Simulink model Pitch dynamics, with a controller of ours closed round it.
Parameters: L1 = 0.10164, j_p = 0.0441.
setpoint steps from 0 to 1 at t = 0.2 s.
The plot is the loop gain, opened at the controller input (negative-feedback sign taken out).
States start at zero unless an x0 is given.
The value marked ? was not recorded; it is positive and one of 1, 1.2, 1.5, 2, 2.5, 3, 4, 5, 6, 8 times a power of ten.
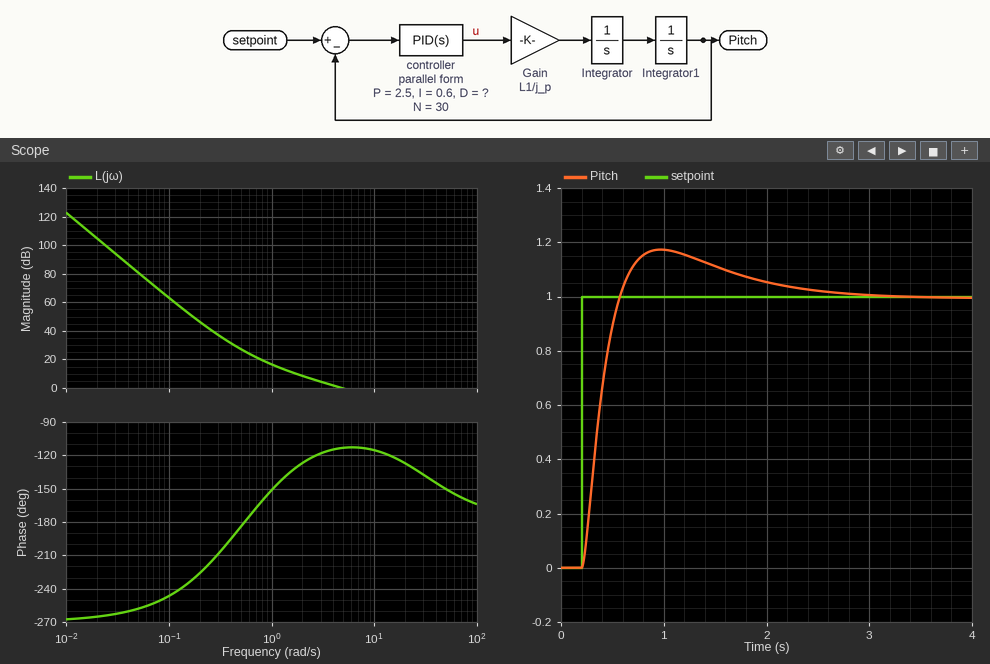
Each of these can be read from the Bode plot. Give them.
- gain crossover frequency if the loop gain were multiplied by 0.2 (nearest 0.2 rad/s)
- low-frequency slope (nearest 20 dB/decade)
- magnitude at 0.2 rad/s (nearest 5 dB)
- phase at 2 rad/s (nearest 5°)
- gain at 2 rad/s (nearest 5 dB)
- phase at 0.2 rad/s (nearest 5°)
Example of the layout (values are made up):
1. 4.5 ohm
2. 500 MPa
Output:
1. 1.2 rad/s
2. -60 dB/decade
3. 45 dB
4. -125°
5. 10 dB
6. -225°
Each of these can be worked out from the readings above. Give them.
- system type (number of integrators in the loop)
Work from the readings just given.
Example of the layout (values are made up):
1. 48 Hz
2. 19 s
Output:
1. 3
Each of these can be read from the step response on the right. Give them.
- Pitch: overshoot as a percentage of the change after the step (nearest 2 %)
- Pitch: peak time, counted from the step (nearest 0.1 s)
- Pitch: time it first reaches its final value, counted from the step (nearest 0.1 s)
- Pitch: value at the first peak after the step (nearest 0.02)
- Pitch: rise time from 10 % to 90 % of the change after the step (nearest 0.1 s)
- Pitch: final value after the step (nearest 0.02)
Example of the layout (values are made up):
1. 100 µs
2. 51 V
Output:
1. 18 %
2. 0.8 s
3. 0.4 s
4. 1.18
5. 0.3 s
6. 1.00
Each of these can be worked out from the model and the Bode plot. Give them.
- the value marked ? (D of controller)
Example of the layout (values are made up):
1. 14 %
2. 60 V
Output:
1. 2
